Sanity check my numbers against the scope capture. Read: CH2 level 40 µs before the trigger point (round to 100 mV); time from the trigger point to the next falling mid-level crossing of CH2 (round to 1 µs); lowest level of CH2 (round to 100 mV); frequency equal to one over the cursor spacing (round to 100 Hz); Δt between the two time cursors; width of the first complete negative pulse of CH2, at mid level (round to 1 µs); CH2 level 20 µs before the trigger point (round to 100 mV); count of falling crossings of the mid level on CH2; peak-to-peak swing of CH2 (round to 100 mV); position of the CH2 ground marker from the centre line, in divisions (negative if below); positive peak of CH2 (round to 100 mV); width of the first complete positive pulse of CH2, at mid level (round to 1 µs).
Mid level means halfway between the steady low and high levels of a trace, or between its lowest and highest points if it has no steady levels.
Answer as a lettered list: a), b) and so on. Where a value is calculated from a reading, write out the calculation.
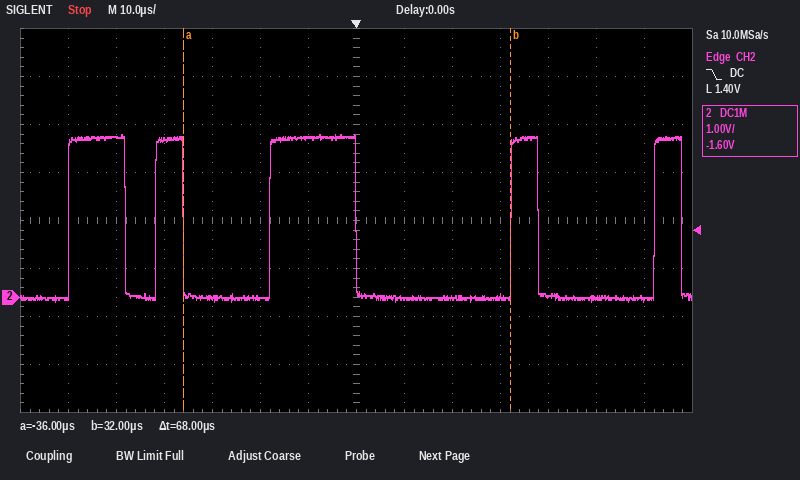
a) 3.3 V
b) 38 µs
c) -100 mV
d) 1 / 68 µs ≈ 14.7 kHz
e) 68 µs
f) 6 µs
g) 0.0 V
h) 5
i) 3.4 V − (-100 mV) = 3.5 V
j) -1.6 div
k) 3.4 V
l) 12 µs
